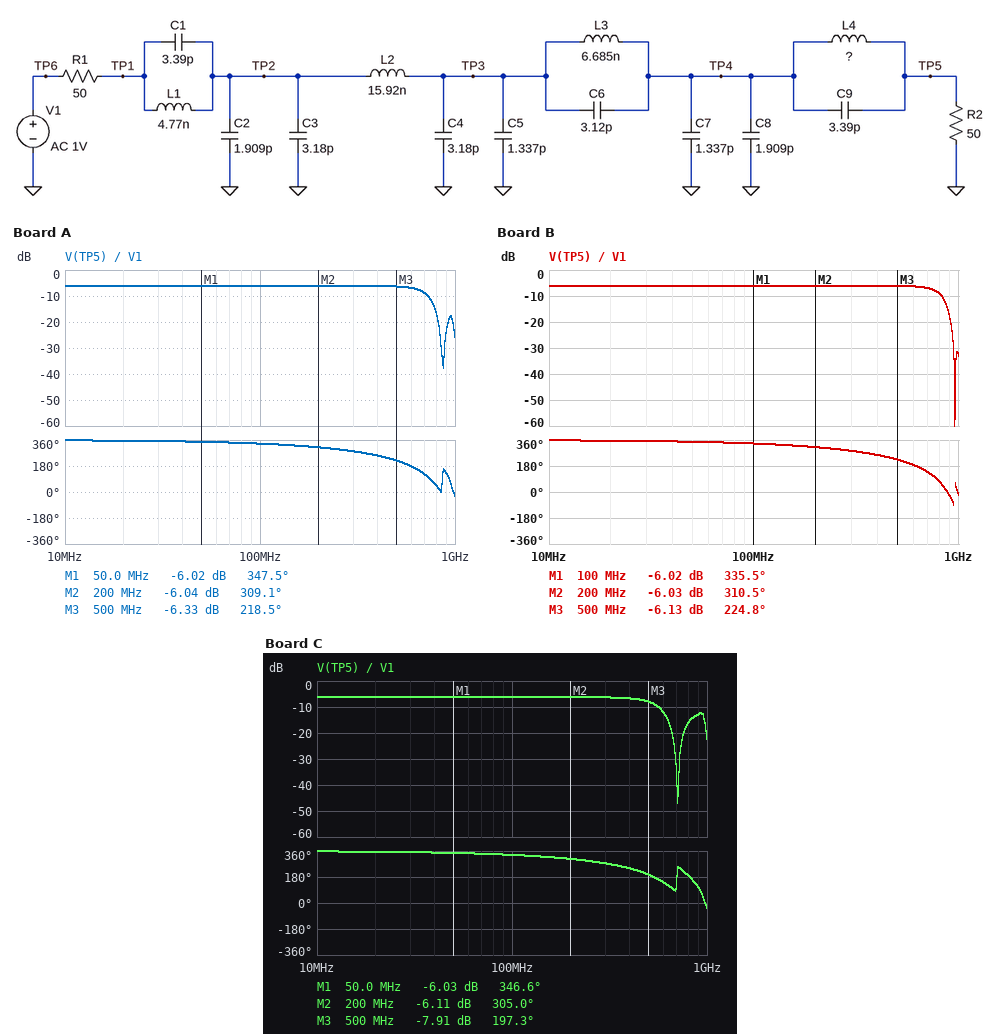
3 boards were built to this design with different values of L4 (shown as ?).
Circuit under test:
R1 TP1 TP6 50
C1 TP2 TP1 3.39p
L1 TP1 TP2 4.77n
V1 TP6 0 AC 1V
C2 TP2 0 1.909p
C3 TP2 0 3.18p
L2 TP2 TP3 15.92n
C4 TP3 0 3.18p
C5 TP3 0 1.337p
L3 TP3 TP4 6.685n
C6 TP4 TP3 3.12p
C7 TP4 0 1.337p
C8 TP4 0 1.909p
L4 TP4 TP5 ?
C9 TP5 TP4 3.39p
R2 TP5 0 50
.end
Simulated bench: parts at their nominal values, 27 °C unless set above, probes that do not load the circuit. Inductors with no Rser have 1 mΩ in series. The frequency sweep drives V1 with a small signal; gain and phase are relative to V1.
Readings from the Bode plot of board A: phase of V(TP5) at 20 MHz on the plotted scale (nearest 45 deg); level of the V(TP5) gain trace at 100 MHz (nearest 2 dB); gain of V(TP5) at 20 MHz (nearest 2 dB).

360 deg
-6 dB
-6 dB
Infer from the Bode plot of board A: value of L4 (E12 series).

10 nH
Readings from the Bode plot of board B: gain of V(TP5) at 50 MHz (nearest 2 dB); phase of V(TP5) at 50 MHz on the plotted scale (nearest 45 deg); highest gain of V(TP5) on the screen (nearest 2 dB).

-6 dB
360 deg
-6 dB
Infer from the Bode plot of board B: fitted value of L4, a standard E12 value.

8.2 nH
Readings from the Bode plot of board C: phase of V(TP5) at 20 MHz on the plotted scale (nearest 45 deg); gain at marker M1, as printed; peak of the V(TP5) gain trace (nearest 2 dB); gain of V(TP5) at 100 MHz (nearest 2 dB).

360 deg
-6.03 dB
-6 dB
-6 dB
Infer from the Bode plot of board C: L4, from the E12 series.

15 nH
